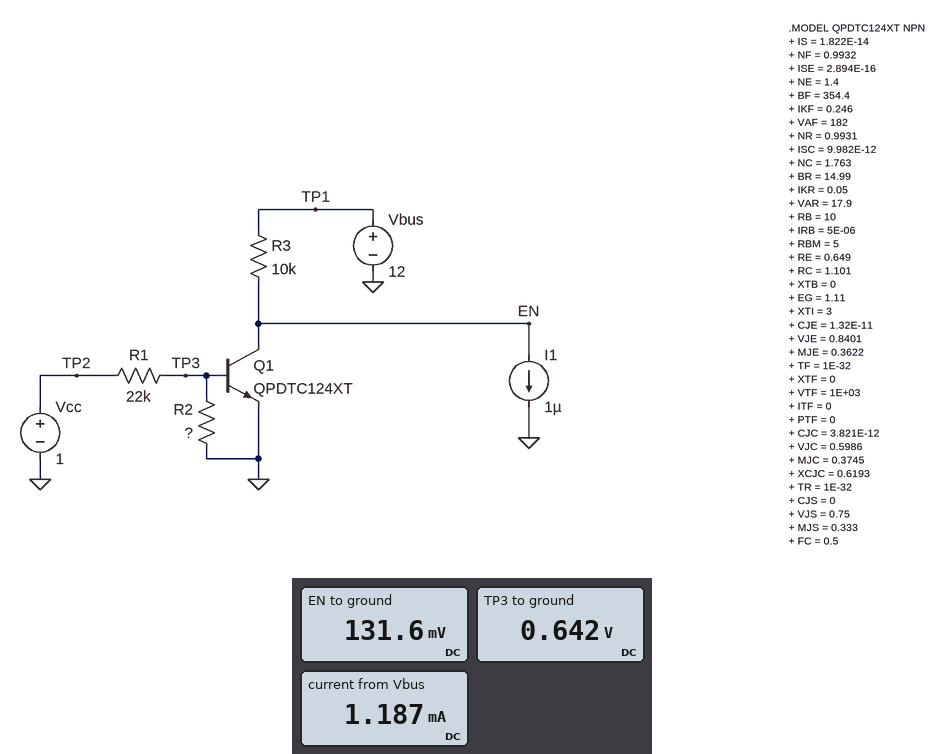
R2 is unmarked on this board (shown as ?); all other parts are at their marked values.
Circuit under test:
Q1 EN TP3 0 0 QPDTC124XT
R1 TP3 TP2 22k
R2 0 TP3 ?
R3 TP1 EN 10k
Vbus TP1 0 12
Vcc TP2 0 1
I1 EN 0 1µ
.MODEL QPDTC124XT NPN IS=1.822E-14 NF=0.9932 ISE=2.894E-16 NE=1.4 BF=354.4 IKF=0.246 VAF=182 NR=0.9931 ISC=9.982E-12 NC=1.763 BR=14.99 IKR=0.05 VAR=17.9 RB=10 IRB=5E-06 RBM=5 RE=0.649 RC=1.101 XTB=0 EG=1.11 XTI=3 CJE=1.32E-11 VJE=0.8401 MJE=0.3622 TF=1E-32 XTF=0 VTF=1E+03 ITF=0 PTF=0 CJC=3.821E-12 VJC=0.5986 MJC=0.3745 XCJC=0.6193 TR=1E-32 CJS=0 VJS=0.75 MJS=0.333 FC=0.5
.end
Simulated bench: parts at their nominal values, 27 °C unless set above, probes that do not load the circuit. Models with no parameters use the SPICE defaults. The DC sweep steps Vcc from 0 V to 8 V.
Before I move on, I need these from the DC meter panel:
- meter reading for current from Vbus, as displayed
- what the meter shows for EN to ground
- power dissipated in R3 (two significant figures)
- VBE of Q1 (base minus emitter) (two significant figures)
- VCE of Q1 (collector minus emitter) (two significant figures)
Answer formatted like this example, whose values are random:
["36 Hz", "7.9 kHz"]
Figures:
["1.187 mA", "131.6 mV", "14 mW", "640 mV", "130 mV"]
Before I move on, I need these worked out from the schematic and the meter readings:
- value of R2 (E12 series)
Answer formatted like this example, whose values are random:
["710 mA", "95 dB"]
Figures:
["56 kΩ"]
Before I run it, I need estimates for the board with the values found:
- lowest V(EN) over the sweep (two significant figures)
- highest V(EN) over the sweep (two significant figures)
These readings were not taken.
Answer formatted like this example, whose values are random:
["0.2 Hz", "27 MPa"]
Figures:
["11 mV", "12 V"]
